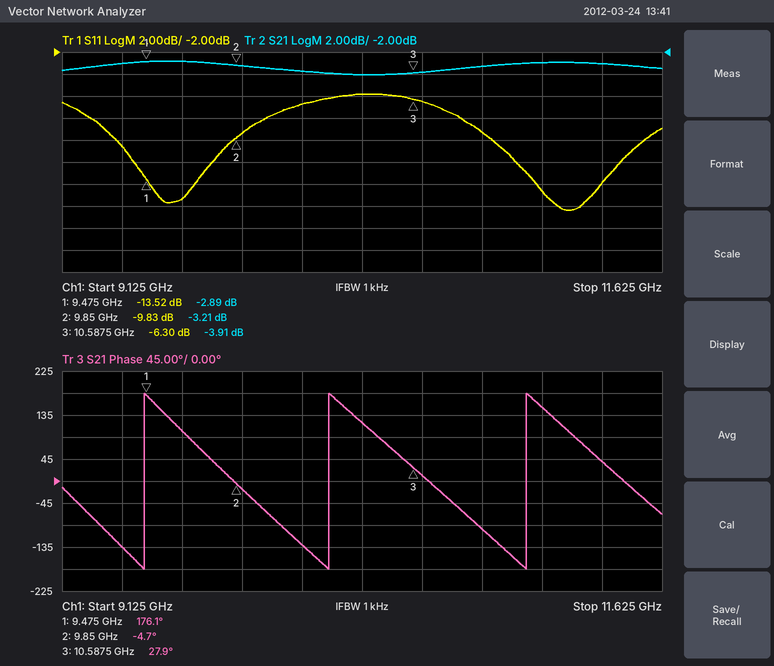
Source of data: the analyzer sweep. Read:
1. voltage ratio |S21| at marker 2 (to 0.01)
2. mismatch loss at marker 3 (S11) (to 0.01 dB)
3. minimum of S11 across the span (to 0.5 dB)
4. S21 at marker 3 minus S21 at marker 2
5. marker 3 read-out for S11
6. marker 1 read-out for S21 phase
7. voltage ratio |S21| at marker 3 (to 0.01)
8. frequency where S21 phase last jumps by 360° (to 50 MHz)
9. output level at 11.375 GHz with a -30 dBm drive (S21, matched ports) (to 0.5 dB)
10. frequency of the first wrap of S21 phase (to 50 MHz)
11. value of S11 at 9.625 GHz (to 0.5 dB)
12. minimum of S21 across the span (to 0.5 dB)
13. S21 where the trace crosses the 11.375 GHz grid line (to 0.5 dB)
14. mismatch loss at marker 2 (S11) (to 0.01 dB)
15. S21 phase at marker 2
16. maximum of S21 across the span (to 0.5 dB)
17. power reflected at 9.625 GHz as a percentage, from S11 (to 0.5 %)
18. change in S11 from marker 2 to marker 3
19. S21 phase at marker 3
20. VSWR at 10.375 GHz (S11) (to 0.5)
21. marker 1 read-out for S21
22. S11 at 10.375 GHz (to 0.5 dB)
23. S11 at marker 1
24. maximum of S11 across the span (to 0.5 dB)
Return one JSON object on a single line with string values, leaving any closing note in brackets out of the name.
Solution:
{"voltage ratio |S21| at marker 2": "0.69", "mismatch loss at marker 3 (S11)": "1.16 dB", "minimum of S11 across the span": "-16.5 dB", "S21 at marker 3 minus S21 at marker 2": "-0.70 dB", "marker 3 read-out for S11": "-6.30 dB", "marker 1 read-out for S21 phase": "176.1°", "voltage ratio |S21| at marker 3": "0.64", "frequency where S21 phase last jumps by 360°": "11.05 GHz", "output level at 11.375 GHz with a -30 dBm drive (S21, matched ports)": "-33.0 dBm", "frequency of the first wrap of S21 phase": "9.45 GHz", "value of S11 at 9.625 GHz": "-15.5 dB", "minimum of S21 across the span": "-4.0 dB", "S21 where the trace crosses the 11.375 GHz grid line": "-3.0 dB", "mismatch loss at marker 2 (S11)": "0.48 dB", "S21 phase at marker 2": "-4.7°", "maximum of S21 across the span": "-3.0 dB", "power reflected at 9.625 GHz as a percentage, from S11": "3.0 %", "change in S11 from marker 2 to marker 3": "3.53 dB", "S21 phase at marker 3": "27.9°", "VSWR at 10.375 GHz (S11)": "3.0", "marker 1 read-out for S21": "-2.89 dB", "S11 at 10.375 GHz": "-6.0 dB", "S11 at marker 1": "-13.52 dB", "maximum of S11 across the span": "-6.0 dB"}
